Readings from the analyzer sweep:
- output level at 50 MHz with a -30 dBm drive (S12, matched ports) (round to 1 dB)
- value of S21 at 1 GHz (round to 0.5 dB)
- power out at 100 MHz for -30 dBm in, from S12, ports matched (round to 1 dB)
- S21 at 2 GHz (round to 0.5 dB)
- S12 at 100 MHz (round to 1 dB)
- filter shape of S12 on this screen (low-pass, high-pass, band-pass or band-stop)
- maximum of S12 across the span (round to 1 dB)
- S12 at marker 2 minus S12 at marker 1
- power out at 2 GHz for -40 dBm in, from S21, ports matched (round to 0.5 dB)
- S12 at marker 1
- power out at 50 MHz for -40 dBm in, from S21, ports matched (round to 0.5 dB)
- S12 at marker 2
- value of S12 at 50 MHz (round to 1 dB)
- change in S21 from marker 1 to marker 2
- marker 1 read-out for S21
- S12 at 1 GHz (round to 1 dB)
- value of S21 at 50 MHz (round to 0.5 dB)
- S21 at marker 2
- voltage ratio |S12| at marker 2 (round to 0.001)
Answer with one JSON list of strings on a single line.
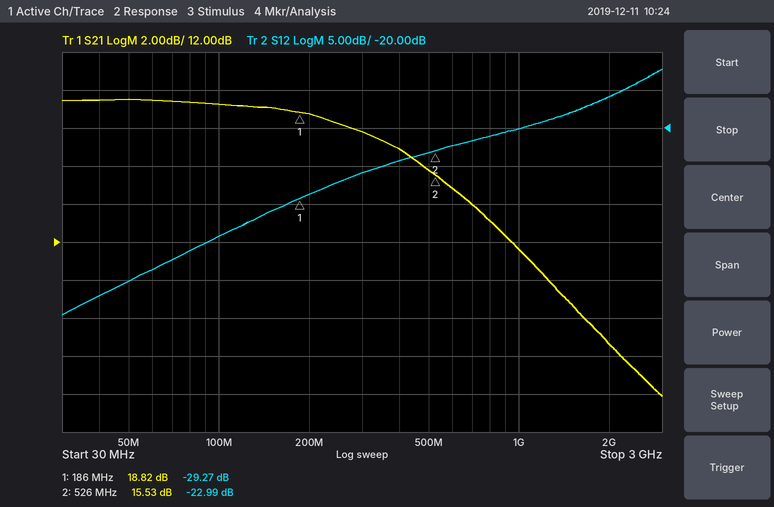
["-70 dBm", "11.5 dB", "-64 dBm", "6.5 dB", "-34 dB", "high-pass", "-12 dB", "6.28 dB", "-33.5 dBm", "-29.27 dB", "-20.5 dBm", "-22.99 dB", "-40 dB", "-3.29 dB", "18.82 dB", "-20 dB", "19.5 dB", "15.53 dB", "0.071"]
